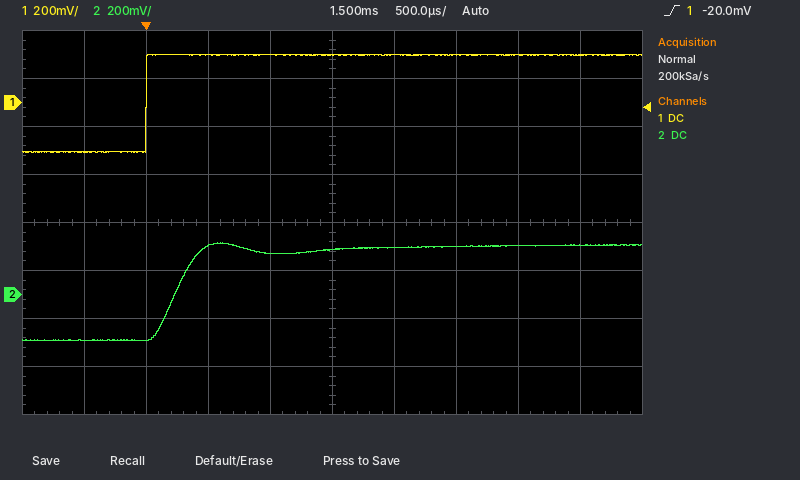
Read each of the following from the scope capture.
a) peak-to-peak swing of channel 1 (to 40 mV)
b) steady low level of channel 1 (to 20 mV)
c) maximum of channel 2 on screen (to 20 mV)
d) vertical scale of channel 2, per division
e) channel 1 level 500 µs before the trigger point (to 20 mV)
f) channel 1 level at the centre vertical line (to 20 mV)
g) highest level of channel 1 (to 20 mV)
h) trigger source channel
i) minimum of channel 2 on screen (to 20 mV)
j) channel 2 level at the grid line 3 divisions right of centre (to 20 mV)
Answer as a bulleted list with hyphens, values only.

- 400 mV
- -200 mV
- 220 mV
- 200 mV
- -200 mV
- 200 mV
- 200 mV
- channel 1
- -200 mV
- 200 mV
